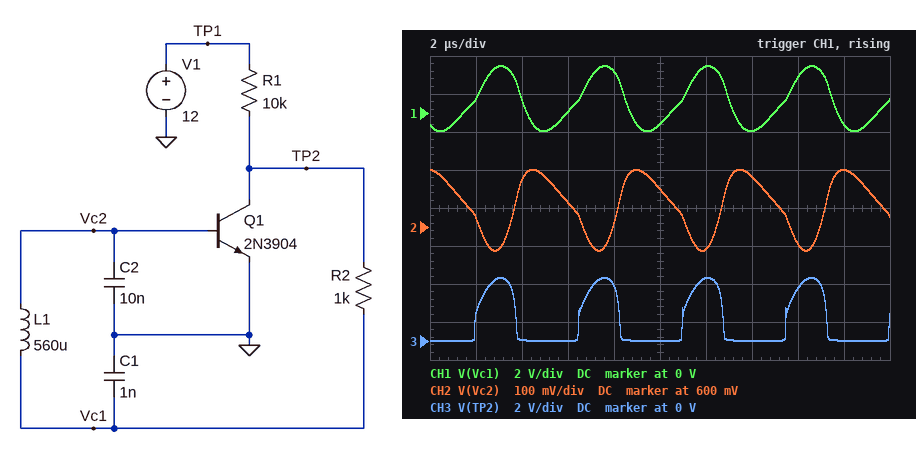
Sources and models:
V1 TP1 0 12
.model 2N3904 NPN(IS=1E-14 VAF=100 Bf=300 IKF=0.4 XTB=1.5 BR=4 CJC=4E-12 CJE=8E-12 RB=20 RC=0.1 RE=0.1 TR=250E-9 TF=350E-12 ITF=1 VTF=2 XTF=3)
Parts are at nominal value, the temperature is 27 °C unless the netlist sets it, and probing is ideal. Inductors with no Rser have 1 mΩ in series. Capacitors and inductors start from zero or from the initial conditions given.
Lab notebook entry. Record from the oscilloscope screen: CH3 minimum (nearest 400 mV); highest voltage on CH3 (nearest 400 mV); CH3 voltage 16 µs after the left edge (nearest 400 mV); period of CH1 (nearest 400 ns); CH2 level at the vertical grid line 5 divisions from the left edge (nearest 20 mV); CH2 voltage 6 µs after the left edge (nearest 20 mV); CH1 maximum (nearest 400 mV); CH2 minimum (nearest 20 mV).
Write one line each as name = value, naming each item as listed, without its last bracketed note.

CH3 minimum = 0 V
highest voltage on CH3 = 3.2 V
CH3 voltage 16 µs after the left edge = 2.8 V
period of CH1 = 4.4 µs
CH2 level at the vertical grid line 5 divisions from the left edge = 700 mV
CH2 voltage 6 µs after the left edge = 660 mV
CH1 maximum = 2.4 V
CH2 minimum = 540 mV
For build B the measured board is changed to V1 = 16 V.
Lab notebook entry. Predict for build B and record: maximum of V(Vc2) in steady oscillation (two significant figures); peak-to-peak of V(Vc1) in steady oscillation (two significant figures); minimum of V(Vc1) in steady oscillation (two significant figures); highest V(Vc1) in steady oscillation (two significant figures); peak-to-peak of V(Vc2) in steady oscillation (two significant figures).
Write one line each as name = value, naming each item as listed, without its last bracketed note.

maximum of V(Vc2) in steady oscillation = 770 mV
peak-to-peak of V(Vc1) in steady oscillation = 4.1 V
minimum of V(Vc1) in steady oscillation = -1.2 V
highest V(Vc1) in steady oscillation = 2.8 V
peak-to-peak of V(Vc2) in steady oscillation = 230 mV
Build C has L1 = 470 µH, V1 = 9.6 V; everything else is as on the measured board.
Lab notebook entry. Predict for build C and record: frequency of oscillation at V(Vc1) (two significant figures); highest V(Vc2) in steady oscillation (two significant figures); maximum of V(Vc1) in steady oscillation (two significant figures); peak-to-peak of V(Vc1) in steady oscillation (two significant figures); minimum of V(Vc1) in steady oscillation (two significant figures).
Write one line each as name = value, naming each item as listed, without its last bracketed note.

frequency of oscillation at V(Vc1) = 240 kHz
highest V(Vc2) in steady oscillation = 740 mV
maximum of V(Vc1) in steady oscillation = 2.2 V
peak-to-peak of V(Vc1) in steady oscillation = 3.0 V
minimum of V(Vc1) in steady oscillation = -810 mV
